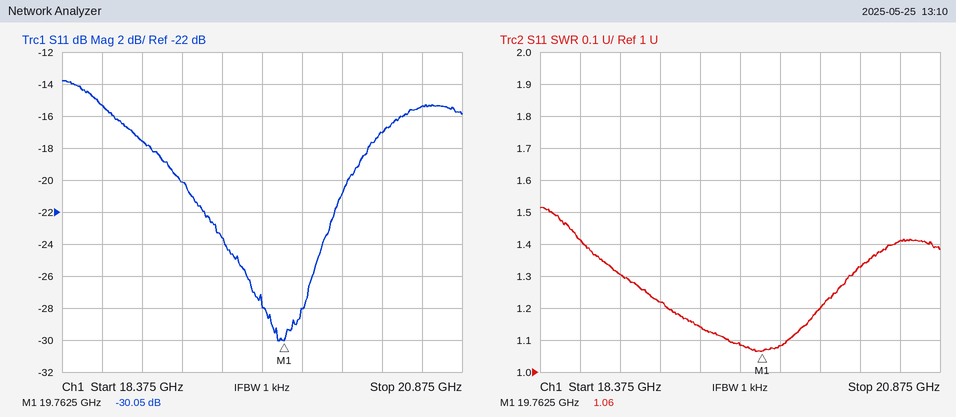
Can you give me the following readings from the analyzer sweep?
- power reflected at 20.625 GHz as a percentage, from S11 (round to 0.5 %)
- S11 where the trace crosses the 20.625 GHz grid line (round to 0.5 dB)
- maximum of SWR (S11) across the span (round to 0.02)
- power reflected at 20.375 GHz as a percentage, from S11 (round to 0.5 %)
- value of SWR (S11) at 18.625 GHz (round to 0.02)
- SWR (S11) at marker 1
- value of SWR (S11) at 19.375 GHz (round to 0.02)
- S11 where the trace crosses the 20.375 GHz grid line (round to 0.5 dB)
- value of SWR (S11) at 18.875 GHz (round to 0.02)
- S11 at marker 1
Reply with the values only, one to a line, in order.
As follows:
3.0 %
-15.5 dB
1.52
2.0 %
1.42
1.06
1.14
-17.0 dB
1.30
-30.05 dB
